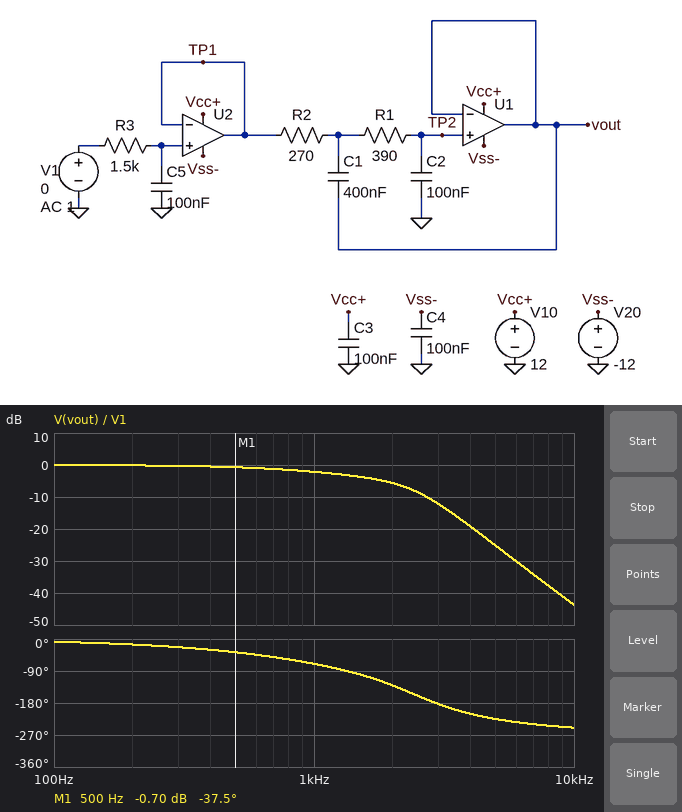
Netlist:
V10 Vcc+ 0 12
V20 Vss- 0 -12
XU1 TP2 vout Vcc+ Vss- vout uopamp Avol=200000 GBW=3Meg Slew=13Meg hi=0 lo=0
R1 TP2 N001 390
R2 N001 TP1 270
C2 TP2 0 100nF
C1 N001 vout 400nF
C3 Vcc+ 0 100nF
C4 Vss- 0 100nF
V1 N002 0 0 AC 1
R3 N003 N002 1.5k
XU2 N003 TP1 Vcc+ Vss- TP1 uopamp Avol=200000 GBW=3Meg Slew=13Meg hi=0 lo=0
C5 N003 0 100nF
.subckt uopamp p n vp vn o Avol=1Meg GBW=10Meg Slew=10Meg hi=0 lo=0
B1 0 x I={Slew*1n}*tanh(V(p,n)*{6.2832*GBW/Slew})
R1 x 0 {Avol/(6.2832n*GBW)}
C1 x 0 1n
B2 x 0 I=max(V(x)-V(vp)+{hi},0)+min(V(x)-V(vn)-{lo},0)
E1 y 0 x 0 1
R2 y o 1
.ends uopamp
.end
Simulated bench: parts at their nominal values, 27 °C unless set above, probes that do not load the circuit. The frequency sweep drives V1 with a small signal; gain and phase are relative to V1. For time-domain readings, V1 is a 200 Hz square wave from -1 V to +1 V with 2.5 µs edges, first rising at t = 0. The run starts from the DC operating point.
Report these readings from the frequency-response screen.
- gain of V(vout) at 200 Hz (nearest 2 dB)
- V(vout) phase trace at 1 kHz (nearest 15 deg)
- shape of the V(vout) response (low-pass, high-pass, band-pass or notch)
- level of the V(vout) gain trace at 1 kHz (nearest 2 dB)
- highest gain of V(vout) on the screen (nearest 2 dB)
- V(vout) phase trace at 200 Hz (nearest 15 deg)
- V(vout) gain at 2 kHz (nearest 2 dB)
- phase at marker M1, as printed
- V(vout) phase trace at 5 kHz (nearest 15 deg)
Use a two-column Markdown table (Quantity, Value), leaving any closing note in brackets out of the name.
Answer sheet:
| Quantity | Value |
|---|---|
| gain of V(vout) at 200 Hz | 0 dB |
| V(vout) phase trace at 1 kHz | -75 deg |
| shape of the V(vout) response | low-pass |
| level of the V(vout) gain trace at 1 kHz | -2 dB |
| highest gain of V(vout) on the screen | 0 dB |
| V(vout) phase trace at 200 Hz | -15 deg |
| V(vout) gain at 2 kHz | -6 dB |
| phase at marker M1, as printed | -37.5 deg |
| V(vout) phase trace at 5 kHz | -225 deg |
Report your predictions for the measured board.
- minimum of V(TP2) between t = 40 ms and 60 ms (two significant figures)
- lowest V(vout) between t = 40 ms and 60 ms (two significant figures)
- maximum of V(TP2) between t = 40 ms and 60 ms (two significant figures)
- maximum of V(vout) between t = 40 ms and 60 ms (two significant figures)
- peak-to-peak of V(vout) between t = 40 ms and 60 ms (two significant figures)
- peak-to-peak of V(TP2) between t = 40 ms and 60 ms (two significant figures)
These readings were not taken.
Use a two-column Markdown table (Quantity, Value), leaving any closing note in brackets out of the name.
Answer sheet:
| Quantity | Value |
|---|---|
| minimum of V(TP2) between t = 40 ms and 60 ms | -1.0 V |
| lowest V(vout) between t = 40 ms and 60 ms | -1.0 V |
| maximum of V(TP2) between t = 40 ms and 60 ms | 1.0 V |
| maximum of V(vout) between t = 40 ms and 60 ms | 1.0 V |
| peak-to-peak of V(vout) between t = 40 ms and 60 ms | 2.0 V |
| peak-to-peak of V(TP2) between t = 40 ms and 60 ms | 2.0 V |
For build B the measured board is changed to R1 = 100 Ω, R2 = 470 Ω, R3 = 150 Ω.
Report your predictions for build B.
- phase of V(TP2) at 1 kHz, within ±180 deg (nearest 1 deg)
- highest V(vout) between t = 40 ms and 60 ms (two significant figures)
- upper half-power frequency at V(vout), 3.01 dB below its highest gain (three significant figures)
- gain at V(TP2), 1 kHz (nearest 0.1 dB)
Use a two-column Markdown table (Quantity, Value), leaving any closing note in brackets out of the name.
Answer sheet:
| Quantity | Value |
|---|---|
| phase of V(TP2) at 1 kHz, within ±180 deg | -27 deg |
| highest V(vout) between t = 40 ms and 60 ms | 1.1 V |
| upper half-power frequency at V(vout), 3.01 dB below its highest gain | 3.71 kHz |
| gain at V(TP2), 1 kHz | 0 dB |
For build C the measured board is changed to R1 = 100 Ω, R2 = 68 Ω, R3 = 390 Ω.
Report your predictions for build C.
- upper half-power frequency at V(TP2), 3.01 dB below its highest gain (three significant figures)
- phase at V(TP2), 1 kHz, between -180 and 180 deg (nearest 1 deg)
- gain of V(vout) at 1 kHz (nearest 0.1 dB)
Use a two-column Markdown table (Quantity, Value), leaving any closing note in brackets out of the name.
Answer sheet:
| Quantity | Value |
|---|---|
| upper half-power frequency at V(TP2), 3.01 dB below its highest gain | 4.92 kHz |
| phase at V(TP2), 1 kHz, between -180 and 180 deg | -20 deg |
| gain of V(vout) at 1 kHz | -0.2 dB |
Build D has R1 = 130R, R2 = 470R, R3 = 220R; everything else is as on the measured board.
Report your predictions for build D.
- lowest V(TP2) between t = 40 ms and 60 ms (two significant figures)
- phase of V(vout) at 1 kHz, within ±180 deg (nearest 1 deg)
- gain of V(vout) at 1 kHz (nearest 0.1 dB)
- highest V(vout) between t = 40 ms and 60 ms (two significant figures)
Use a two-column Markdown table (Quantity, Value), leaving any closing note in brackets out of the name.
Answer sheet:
| Quantity | Value |
|---|---|
| lowest V(TP2) between t = 40 ms and 60 ms | -1.2 V |
| phase of V(vout) at 1 kHz, within ±180 deg | -31 deg |
| gain of V(vout) at 1 kHz | 0.1 dB |
| highest V(vout) between t = 40 ms and 60 ms | 1.2 V |
